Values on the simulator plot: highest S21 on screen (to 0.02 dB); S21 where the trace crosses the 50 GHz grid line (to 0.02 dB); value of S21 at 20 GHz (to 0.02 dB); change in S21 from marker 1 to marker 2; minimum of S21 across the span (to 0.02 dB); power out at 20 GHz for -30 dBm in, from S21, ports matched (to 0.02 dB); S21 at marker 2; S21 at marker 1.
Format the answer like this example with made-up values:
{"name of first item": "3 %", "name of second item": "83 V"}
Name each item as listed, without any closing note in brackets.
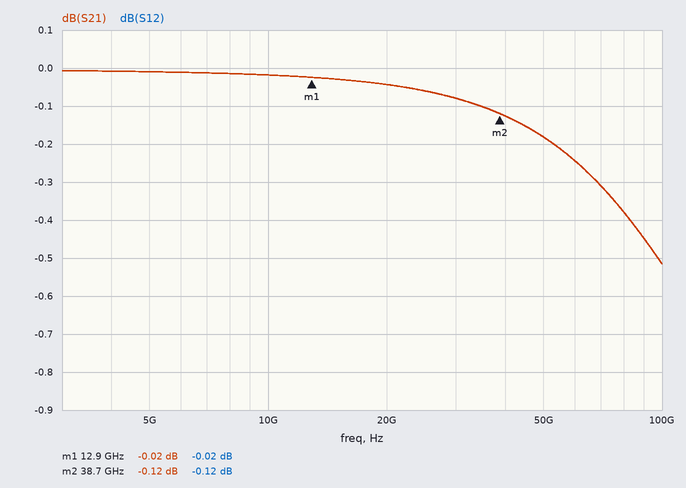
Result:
{"highest S21 on screen": "0.00 dB", "S21 where the trace crosses the 50 GHz grid line": "-0.18 dB", "value of S21 at 20 GHz": "-0.04 dB", "change in S21 from marker 1 to marker 2": "-0.10 dB", "minimum of S21 across the span": "-0.52 dB", "power out at 20 GHz for -30 dBm in, from S21, ports matched": "-30.04 dBm", "S21 at marker 2": "-0.12 dB", "S21 at marker 1": "-0.02 dB"}
